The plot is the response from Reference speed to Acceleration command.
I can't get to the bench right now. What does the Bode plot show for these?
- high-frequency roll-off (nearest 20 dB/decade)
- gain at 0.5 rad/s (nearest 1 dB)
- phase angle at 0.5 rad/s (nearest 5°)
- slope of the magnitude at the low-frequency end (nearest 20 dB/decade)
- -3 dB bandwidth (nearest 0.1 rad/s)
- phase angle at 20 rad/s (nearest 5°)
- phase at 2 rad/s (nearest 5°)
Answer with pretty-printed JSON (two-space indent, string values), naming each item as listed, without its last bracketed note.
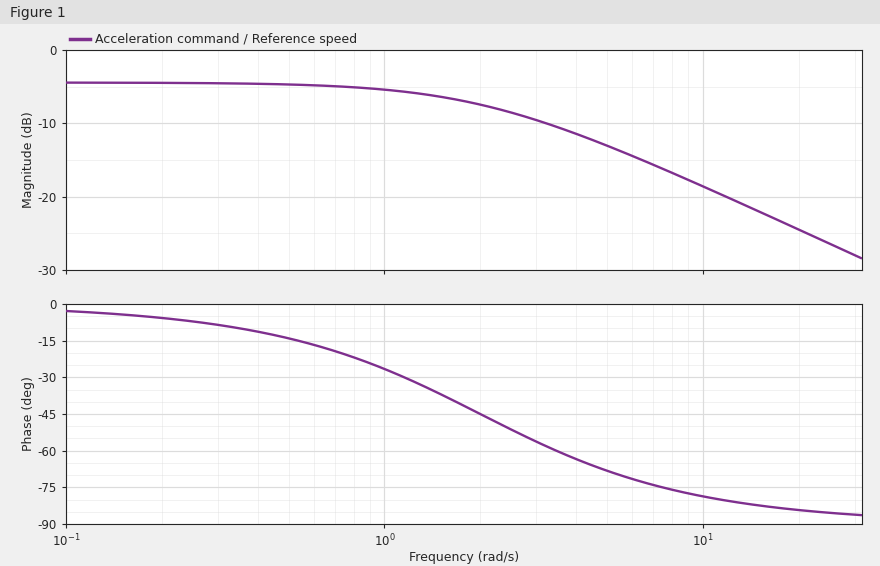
{
  "high-frequency roll-off": "-20 dB/decade",
  "gain at 0.5 rad/s": "-5 dB",
  "phase angle at 0.5 rad/s": "-15°",
  "slope of the magnitude at the low-frequency end": "0 dB/decade",
  "-3 dB bandwidth": "2.0 rad/s",
  "phase angle at 20 rad/s": "-85°",
  "phase at 2 rad/s": "-45°"
}
